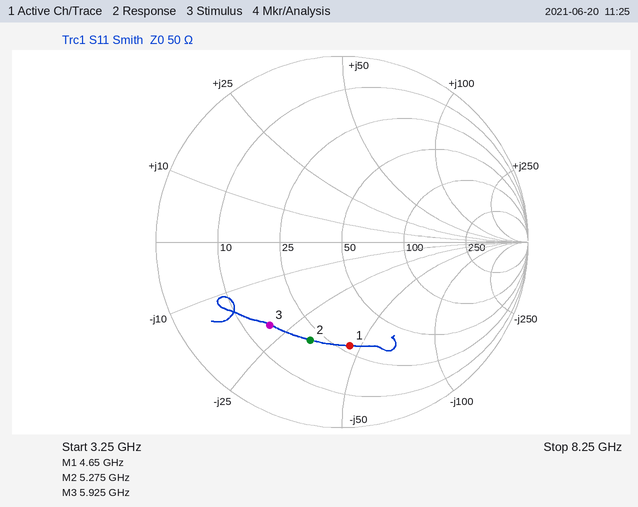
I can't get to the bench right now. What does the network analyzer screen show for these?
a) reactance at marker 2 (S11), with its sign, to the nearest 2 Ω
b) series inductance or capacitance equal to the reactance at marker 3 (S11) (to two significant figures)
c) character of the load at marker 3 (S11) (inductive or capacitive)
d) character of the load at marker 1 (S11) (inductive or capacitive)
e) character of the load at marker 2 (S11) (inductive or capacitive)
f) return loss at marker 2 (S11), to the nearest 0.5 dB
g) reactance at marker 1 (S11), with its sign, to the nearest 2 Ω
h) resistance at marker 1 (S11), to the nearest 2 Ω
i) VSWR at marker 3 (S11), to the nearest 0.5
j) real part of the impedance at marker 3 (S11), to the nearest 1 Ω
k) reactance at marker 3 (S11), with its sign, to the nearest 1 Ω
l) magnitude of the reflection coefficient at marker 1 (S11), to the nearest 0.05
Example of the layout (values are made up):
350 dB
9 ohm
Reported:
-32 Ω
1.3 pF
capacitive
capacitive
capacitive
5.0 dB
-46 Ω
28 Ω
4.0
15 Ω
-21 Ω
0.55
